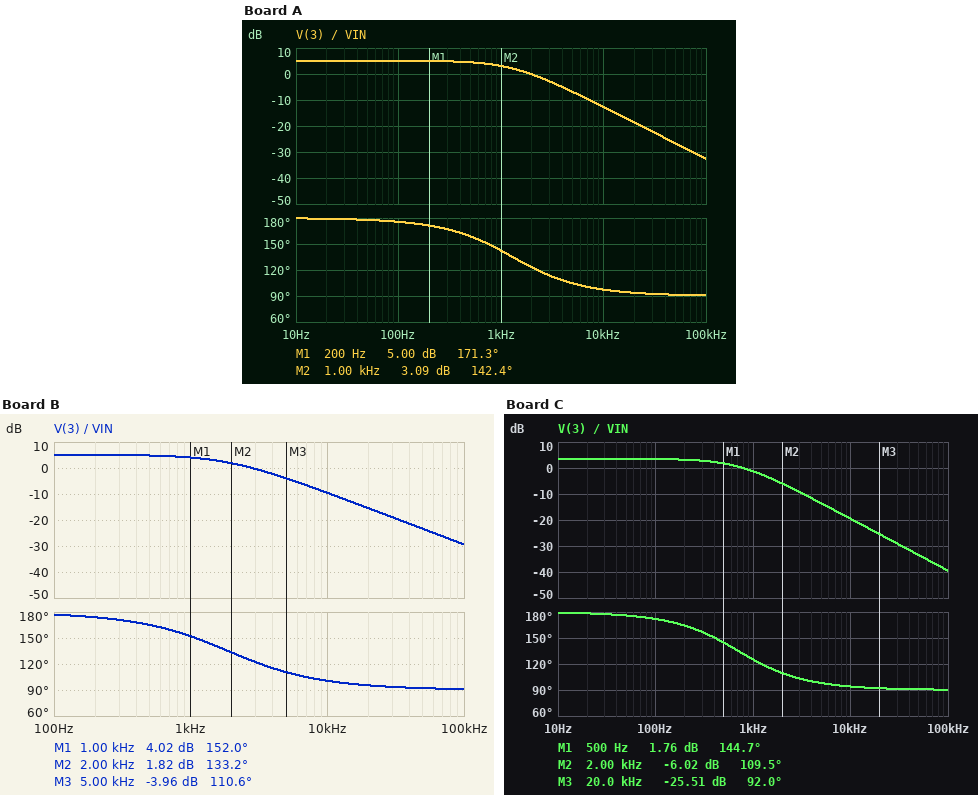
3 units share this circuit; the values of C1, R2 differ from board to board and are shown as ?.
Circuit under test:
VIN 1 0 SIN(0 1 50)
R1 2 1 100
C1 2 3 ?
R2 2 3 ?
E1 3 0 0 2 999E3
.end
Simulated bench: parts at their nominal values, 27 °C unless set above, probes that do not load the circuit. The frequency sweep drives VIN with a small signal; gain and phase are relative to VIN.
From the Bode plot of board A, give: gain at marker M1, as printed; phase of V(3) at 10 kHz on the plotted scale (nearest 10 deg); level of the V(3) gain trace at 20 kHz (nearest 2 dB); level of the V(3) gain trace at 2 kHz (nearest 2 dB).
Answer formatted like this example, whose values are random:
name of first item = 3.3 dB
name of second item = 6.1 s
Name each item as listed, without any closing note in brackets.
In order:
gain at marker M1, as printed = 5.00 dB
phase of V(3) at 10 kHz on the plotted scale = 100 deg
level of the V(3) gain trace at 20 kHz = -18 dB
level of the V(3) gain trace at 2 kHz = 0 dB
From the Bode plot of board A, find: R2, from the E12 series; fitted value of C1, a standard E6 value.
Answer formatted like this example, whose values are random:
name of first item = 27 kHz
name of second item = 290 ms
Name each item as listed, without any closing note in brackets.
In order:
R2, from the E12 series = 180 Ω
fitted value of C1, a standard E6 value = 680 nF
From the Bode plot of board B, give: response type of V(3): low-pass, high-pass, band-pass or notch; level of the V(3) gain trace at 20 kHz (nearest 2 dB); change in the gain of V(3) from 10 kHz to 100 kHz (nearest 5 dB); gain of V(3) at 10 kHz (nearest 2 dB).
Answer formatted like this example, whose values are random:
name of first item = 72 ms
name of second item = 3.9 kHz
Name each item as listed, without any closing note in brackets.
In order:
response type of V(3): low-pass, high-pass, band-pass or notch = low-pass
level of the V(3) gain trace at 20 kHz = -16 dB
change in the gain of V(3) from 10 kHz to 100 kHz = -20 dB
gain of V(3) at 10 kHz = -10 dB
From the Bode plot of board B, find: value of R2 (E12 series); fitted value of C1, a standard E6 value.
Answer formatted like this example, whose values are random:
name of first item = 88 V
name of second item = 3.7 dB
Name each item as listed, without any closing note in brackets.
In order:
value of R2 = 180 Ω
fitted value of C1, a standard E6 value = 470 nF
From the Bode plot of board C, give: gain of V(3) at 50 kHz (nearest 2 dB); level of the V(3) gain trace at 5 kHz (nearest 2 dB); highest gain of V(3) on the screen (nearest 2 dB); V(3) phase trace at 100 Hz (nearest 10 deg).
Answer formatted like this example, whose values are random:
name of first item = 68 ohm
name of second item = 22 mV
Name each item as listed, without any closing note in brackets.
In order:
gain of V(3) at 50 kHz = -34 dB
level of the V(3) gain trace at 5 kHz = -14 dB
highest gain of V(3) on the screen = 4 dB
V(3) phase trace at 100 Hz = 170 deg
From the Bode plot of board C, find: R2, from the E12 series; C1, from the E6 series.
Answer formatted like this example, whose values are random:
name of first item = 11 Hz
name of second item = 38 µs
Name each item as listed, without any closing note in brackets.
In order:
R2, from the E12 series = 150 Ω
C1, from the E6 series = 1.5 µF
